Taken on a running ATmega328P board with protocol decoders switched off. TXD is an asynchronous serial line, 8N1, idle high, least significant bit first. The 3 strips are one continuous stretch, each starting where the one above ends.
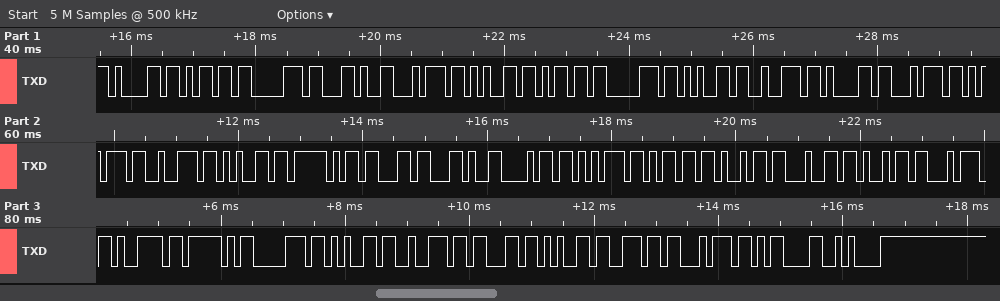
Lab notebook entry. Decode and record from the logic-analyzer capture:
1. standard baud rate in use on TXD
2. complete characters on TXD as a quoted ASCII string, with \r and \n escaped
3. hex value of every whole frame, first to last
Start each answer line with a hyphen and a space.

- 9600 baud
- "amp,temperature_c,humidity_percent\r\n"
- 0x61 0x6D 0x70 0x2C 0x74 0x65 0x6D 0x70 0x65 0x72 0x61 0x74 0x75 0x72 0x65 0x5F 0x63 0x2C 0x68 0x75 0x6D 0x69 0x64 0x69 0x74 0x79 0x5F 0x70 0x65 0x72 0x63 0x65 0x6E 0x74 0x0D 0x0A
